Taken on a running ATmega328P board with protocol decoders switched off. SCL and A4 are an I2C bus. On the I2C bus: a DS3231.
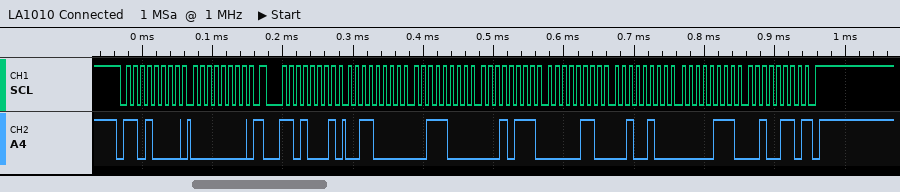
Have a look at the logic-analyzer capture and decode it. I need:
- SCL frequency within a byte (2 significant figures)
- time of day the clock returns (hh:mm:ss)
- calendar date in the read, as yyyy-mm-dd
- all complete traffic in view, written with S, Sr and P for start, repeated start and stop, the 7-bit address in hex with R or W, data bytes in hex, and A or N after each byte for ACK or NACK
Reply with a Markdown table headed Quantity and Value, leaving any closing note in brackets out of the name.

| Quantity | Value |
|---|---|
| SCL frequency within a byte | 100 kHz |
| time of day the clock returns | 17:38:30 |
| calendar date in the read, as yyyy-mm-dd | 2026-07-24 |
| all complete traffic in view, written with S, Sr and P for start, repeated start and stop, the 7-bit address in hex with R or W, data bytes in hex, and A or N after each byte for ACK or NACK | S 68W A 00 A Sr 68R A 30 A 38 A 17 A 06 A 24 A 07 A 26 N P |
